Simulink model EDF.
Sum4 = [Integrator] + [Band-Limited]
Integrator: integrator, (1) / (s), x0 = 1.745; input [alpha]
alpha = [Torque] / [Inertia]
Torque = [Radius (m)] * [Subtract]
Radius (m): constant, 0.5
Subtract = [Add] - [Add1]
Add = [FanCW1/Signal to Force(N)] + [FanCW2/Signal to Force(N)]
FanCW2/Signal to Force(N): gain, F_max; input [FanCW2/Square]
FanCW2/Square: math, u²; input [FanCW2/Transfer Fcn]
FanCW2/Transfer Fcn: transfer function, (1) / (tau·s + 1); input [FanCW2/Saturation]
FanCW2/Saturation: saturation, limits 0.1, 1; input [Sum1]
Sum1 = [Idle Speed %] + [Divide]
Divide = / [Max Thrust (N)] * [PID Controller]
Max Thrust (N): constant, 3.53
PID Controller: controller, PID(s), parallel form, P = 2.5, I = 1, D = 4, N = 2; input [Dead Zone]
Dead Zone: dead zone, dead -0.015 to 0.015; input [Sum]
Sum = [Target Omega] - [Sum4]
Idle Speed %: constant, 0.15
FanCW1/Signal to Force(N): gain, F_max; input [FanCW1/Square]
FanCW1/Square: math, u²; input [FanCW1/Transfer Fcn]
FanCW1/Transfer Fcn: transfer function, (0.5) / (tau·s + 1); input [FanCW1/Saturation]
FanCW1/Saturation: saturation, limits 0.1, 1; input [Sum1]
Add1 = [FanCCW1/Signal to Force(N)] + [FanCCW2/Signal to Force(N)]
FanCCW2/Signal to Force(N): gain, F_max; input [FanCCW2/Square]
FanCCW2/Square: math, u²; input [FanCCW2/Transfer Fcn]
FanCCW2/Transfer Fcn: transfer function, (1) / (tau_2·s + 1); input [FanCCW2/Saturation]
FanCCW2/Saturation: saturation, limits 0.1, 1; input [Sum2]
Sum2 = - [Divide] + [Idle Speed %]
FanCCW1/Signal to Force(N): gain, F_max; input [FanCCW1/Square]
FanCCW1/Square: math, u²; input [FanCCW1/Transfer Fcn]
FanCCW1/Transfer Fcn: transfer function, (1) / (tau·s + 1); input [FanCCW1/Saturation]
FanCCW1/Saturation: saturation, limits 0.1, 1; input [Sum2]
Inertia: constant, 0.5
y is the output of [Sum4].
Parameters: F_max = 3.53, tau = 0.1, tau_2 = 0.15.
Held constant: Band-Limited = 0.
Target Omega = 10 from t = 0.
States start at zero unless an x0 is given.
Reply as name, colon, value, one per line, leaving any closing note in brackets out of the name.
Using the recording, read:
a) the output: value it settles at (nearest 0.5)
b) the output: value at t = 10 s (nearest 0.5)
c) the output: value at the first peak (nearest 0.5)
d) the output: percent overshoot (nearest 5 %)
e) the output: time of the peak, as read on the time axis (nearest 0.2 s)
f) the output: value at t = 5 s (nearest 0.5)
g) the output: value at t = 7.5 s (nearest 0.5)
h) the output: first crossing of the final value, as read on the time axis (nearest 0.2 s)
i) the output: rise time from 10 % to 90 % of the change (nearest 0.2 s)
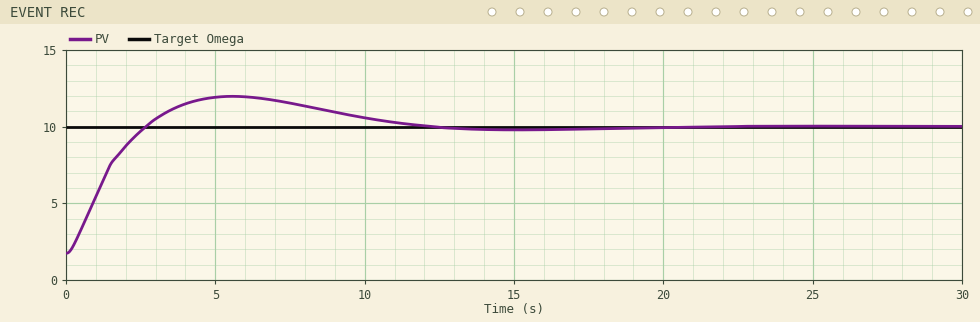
the output: value it settles at: 10.0
the output: value at t = 10 s: 10.5
the output: value at the first peak: 12.0
the output: percent overshoot: 25 %
the output: time of the peak, as read on the time axis: 5.6 s
the output: value at t = 5 s: 12.0
the output: value at t = 7.5 s: 11.5
the output: first crossing of the final value, as read on the time axis: 2.6 s
the output: rise time from 10 % to 90 % of the change: 1.8 s
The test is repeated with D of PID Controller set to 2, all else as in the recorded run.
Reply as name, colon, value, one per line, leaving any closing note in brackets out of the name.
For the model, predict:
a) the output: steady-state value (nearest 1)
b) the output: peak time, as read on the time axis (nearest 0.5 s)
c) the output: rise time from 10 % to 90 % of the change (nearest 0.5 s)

the output: steady-state value: 10
the output: peak time, as read on the time axis: 4.5 s
the output: rise time from 10 % to 90 % of the change: 1.5 s
